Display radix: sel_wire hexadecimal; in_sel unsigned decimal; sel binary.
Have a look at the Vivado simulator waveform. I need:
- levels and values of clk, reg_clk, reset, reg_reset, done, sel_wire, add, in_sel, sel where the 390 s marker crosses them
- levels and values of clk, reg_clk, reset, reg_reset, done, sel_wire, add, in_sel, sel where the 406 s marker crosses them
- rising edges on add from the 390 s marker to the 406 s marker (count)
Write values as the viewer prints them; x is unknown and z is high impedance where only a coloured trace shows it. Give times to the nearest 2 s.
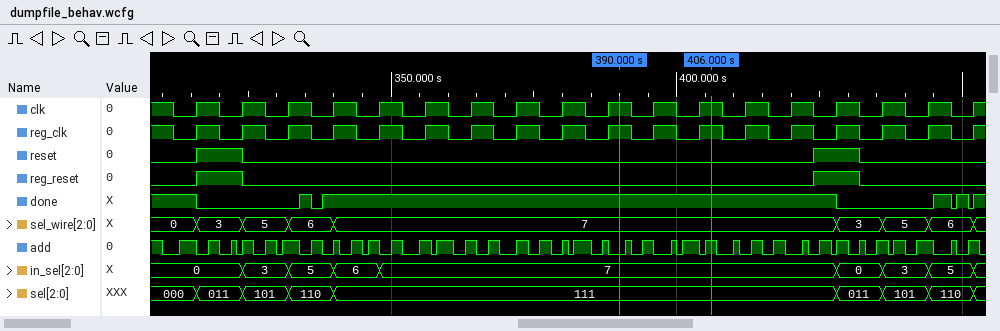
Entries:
clk=1, reg_clk=1, reset=0, reg_reset=0, done=1, sel_wire=7, add=0, in_sel=7, sel=111
clk=1, reg_clk=1, reset=0, reg_reset=0, done=1, sel_wire=7, add=1, in_sel=7, sel=111
5
